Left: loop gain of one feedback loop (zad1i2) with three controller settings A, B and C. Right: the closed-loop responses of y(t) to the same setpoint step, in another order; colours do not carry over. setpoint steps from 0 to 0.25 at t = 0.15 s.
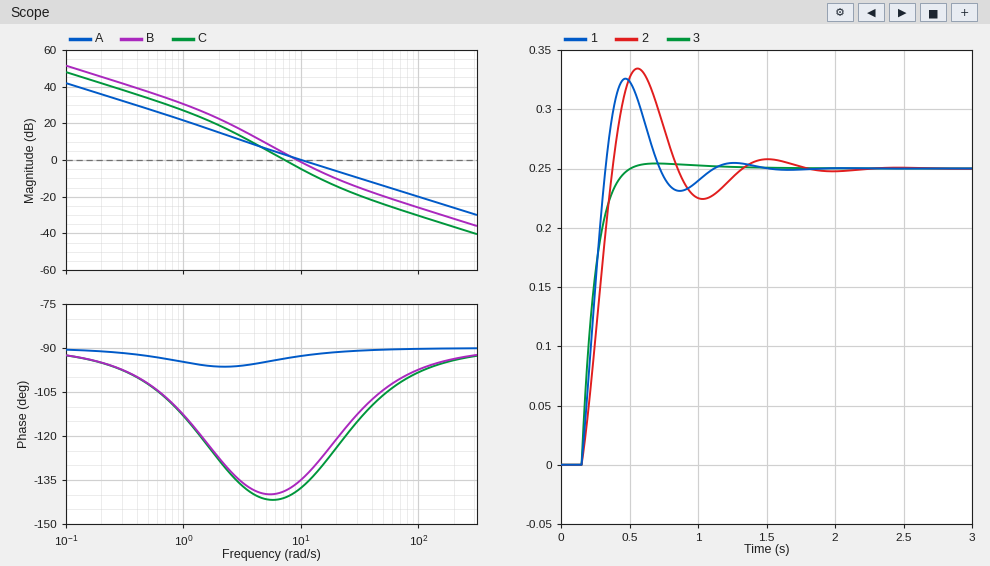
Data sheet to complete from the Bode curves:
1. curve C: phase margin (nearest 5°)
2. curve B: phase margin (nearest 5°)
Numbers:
40°
45°
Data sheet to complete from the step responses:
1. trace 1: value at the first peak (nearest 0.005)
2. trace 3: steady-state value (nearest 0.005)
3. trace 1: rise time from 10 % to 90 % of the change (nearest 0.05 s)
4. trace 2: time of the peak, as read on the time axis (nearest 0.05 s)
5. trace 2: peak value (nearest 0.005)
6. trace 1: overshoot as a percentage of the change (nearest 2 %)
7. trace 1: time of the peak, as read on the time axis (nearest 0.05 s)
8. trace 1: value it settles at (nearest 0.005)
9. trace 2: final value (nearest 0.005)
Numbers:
0.325
0.250
0.15 s
0.55 s
0.335
30 %
0.45 s
0.250
0.250
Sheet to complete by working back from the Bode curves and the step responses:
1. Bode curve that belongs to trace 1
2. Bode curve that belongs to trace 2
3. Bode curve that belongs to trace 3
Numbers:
B
C
A
